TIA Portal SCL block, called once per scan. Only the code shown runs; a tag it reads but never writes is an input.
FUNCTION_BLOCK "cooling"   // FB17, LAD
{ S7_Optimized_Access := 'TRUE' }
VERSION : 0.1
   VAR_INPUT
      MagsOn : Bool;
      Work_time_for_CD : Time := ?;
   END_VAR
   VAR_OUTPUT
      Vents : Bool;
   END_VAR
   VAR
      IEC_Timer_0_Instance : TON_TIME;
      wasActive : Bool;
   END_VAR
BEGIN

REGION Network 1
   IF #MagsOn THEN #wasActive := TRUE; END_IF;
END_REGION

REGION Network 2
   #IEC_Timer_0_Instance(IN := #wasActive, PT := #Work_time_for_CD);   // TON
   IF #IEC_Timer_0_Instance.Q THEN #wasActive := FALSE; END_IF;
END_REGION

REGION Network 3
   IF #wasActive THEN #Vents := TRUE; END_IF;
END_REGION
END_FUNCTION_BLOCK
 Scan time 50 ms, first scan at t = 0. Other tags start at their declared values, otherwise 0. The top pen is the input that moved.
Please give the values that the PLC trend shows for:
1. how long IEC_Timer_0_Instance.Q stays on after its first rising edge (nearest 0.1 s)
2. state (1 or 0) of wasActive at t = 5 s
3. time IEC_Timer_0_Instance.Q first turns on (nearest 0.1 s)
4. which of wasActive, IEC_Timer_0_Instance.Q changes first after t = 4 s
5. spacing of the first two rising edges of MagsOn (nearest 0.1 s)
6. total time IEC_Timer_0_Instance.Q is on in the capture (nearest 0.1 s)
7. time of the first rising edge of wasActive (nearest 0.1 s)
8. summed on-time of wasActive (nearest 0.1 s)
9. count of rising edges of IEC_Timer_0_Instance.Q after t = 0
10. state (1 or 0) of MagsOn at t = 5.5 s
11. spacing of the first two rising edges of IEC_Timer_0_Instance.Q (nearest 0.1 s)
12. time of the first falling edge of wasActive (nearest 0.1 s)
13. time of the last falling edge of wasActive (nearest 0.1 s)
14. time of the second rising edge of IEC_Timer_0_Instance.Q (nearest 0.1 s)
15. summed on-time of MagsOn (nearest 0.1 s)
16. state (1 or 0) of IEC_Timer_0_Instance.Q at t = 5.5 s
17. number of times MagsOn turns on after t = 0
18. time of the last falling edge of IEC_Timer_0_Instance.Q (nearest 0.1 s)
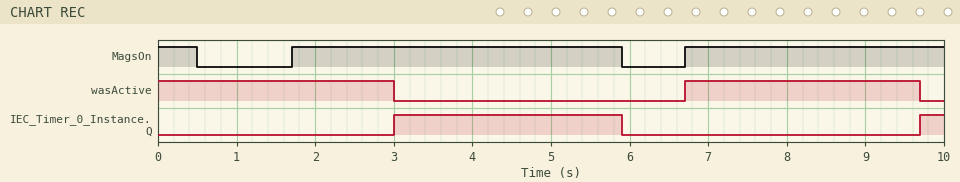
2.9 s
0
3.0 s
IEC_Timer_0_Instance.Q
5.0 s
3.2 s
6.7 s
6.0 s
2
1
6.7 s
3.0 s
9.7 s
9.7 s
8.0 s
1
2
5.9 s
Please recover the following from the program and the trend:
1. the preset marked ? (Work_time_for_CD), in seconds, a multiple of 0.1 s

3.0 s
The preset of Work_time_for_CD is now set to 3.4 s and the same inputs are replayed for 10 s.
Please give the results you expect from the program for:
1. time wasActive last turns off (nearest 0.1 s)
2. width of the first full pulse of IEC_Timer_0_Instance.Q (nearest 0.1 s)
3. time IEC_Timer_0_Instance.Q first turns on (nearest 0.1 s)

3.4 s
2.5 s
3.4 s
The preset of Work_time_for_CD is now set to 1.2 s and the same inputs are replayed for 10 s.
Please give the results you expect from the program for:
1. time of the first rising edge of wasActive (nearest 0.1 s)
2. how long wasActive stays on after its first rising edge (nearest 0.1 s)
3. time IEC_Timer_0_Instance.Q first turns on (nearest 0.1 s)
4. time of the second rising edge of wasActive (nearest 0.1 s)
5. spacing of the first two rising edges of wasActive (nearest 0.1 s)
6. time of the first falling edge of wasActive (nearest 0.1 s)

1.7 s
1.2 s
1.2 s
6.7 s
5.0 s
1.2 s
